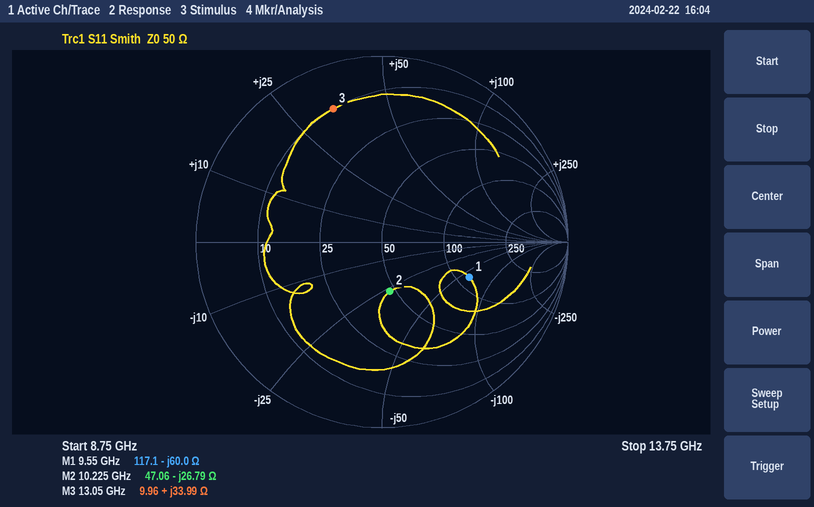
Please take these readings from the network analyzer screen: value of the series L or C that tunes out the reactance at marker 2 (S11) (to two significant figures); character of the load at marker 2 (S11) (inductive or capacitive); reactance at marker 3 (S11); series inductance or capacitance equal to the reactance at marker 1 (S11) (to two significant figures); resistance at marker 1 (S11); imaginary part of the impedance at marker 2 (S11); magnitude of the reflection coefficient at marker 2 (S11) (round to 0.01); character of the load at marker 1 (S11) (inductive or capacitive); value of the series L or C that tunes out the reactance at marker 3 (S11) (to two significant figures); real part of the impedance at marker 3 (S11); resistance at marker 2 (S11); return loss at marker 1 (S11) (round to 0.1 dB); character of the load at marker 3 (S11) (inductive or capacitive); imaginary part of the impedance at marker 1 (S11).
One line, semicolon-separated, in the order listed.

420 pH; capacitive; +33.99 Ω; 280 fF; 117.1 Ω; -26.79 Ω; 0.27; capacitive; 360 fF; 9.96 Ω; 47.06 Ω; 5.9 dB; inductive; -60.0 Ω
